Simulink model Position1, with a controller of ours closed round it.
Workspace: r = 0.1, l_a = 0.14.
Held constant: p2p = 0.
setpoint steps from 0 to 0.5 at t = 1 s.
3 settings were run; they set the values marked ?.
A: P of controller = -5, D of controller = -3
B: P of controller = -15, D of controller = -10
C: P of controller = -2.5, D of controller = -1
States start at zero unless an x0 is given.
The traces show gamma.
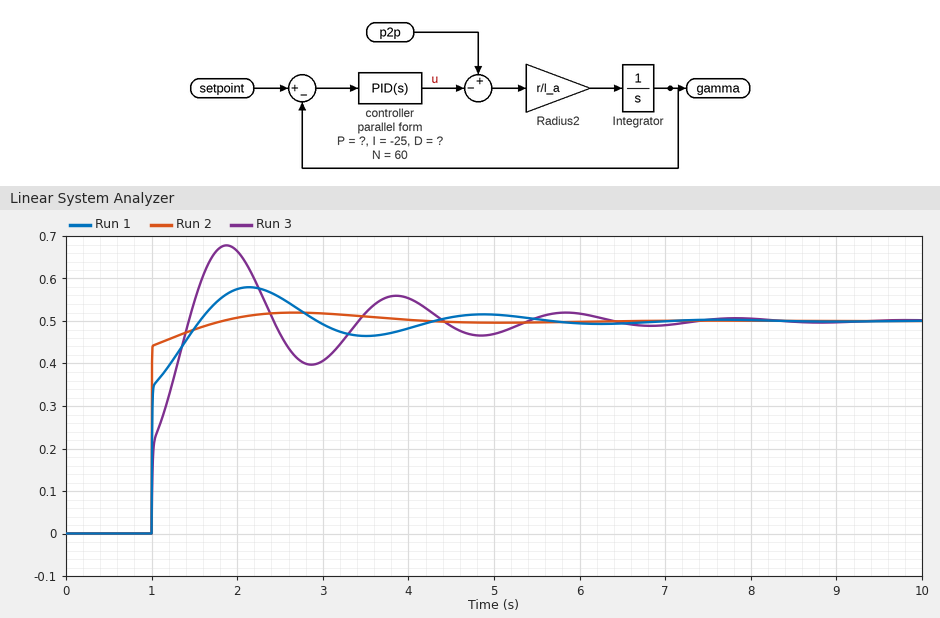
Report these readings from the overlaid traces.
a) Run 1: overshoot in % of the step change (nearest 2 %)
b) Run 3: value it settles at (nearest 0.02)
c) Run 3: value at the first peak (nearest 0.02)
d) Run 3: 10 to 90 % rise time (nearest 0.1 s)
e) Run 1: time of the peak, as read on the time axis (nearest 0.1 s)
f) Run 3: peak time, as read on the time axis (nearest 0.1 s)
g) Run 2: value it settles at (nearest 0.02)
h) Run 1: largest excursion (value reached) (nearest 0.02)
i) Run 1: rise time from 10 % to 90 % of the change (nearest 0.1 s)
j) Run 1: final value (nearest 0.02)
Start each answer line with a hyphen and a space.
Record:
- 16 %
- 0.50
- 0.68
- 0.4 s
- 2.1 s
- 1.9 s
- 0.50
- 0.58
- 0.4 s
- 0.50
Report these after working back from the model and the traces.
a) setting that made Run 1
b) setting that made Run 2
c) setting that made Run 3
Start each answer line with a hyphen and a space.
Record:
- A
- B
- C
